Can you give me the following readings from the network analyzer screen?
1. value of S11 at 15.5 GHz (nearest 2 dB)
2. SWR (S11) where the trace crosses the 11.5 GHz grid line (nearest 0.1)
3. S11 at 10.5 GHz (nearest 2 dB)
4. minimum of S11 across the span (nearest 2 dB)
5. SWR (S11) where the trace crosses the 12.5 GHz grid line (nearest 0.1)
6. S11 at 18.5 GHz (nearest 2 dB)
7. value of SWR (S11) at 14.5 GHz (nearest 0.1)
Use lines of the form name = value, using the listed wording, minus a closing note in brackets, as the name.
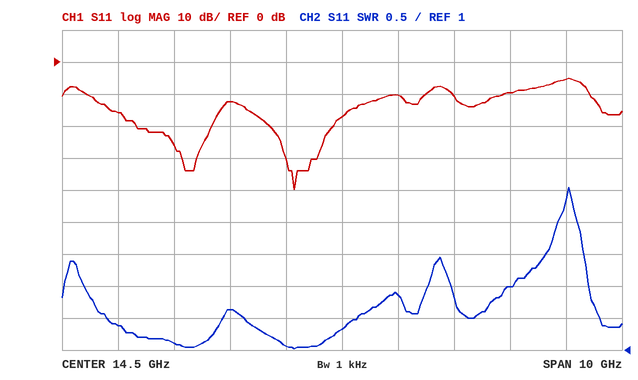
value of S11 at 15.5 GHz = -10 dB
SWR (S11) where the trace crosses the 11.5 GHz grid line = 1.1
S11 at 10.5 GHz = -16 dB
minimum of S11 across the span = -40 dB
SWR (S11) where the trace crosses the 12.5 GHz grid line = 1.6
S11 at 18.5 GHz = -6 dB
value of SWR (S11) at 14.5 GHz = 1.3
